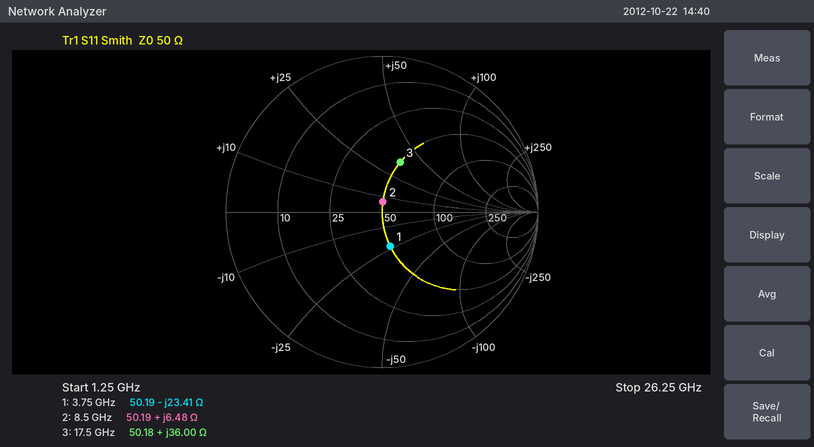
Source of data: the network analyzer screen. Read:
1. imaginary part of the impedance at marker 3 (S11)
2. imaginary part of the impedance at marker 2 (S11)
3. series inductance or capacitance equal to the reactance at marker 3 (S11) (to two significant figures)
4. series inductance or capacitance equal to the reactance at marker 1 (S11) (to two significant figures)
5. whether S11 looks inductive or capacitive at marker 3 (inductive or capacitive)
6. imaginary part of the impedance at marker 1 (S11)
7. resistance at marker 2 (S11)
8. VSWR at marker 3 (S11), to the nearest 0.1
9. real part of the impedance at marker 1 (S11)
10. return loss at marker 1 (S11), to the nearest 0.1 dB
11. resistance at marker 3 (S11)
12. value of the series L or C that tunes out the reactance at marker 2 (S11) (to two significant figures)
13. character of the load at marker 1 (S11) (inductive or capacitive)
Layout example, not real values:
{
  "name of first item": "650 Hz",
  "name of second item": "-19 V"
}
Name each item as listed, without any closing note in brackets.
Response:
{
  "imaginary part of the impedance at marker 3": "+36.00 Ω",
  "imaginary part of the impedance at marker 2": "+6.48 Ω",
  "series inductance or capacitance equal to the reactance at marker 3 (S11)": "330 pH",
  "series inductance or capacitance equal to the reactance at marker 1 (S11)": "1.8 pF",
  "whether S11 looks inductive or capacitive at marker 3": "inductive",
  "imaginary part of the impedance at marker 1": "-23.41 Ω",
  "resistance at marker 2": "50.19 Ω",
  "VSWR at marker 3 (S11), to the nearest 0.1": "2.0",
  "real part of the impedance at marker 1": "50.19 Ω",
  "return loss at marker 1 (S11), to the nearest 0.1 dB": "12.9 dB",
  "resistance at marker 3": "50.18 Ω",
  "value of the series L or C that tunes out the reactance at marker 2 (S11)": "2.9 pF",
  "character of the load at marker 1 (S11)": "capacitive"
}
